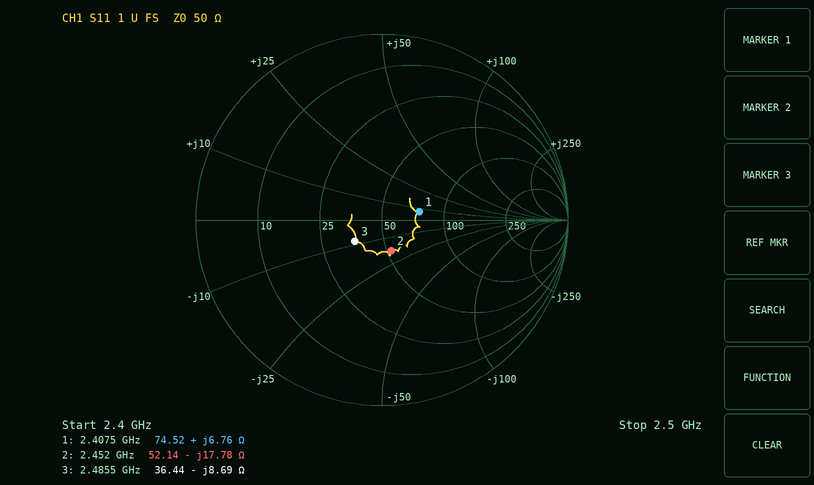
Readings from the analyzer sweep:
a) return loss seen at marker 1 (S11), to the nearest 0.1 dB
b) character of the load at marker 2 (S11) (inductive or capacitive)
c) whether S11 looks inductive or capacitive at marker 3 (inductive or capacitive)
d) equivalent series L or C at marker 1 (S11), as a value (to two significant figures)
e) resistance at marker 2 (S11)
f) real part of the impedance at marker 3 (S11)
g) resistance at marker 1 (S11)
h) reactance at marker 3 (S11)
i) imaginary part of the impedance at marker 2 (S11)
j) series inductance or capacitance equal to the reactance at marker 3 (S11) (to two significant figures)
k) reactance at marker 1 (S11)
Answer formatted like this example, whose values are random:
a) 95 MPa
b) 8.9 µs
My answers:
a) 13.8 dB
b) capacitive
c) capacitive
d) 450 pH
e) 52.14 Ω
f) 36.44 Ω
g) 74.52 Ω
h) -8.69 Ω
i) -17.78 Ω
j) 7.4 pF
k) +6.76 Ω
